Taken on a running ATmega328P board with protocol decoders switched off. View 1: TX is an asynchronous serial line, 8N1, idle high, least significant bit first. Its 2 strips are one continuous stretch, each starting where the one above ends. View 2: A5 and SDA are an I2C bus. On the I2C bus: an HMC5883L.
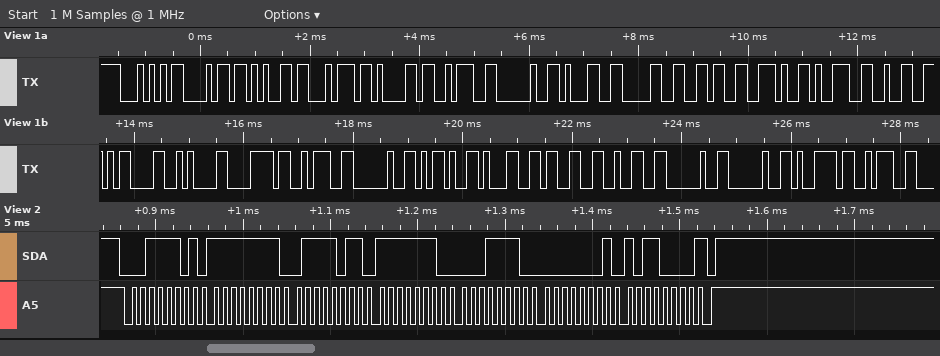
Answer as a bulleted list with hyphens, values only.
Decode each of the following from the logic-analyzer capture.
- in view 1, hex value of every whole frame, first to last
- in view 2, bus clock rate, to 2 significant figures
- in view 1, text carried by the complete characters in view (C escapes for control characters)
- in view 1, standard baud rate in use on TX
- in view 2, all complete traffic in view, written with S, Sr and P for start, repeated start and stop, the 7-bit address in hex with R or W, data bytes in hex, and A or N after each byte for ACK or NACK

- 0x54 0x68 0x65 0x74 0x61 0x3A 0x20 0x31 0x30 0x36 0x2E 0x39 0x32 0x0D 0x0A 0x78 0x3A 0x20 0x2D 0x31 0x33 0x32 0x20 0x20 0x79 0x3A
- 100 kHz
- "Theta: 106.92\r\nx: -132  y:"
- 9600 baud
- S 1ER A FF A 7B A FE A 1E A 01 A B0 N P
